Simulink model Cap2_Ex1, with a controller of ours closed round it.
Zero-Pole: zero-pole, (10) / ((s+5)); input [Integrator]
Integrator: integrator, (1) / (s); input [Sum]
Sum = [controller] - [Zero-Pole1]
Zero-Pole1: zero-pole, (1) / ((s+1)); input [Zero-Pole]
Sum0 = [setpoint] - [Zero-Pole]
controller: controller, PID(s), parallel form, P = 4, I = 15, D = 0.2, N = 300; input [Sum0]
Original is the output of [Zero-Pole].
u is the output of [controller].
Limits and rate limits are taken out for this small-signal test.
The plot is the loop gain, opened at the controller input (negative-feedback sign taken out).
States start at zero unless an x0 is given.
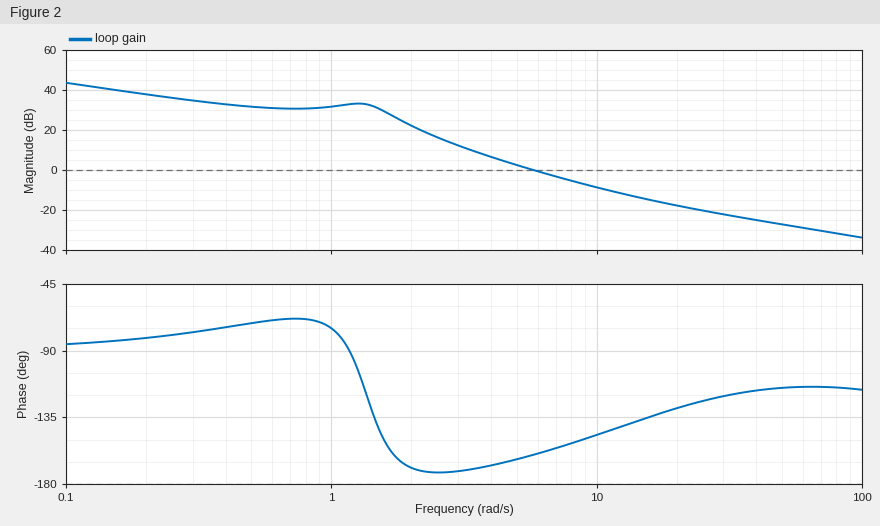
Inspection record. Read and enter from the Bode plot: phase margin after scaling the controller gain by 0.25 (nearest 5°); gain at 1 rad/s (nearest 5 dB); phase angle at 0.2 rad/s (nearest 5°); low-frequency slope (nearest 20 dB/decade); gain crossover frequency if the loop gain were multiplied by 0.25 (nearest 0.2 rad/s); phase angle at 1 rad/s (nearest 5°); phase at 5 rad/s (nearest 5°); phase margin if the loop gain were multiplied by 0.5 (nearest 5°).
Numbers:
10°
30 dB
-80°
-20 dB/decade
3.0 rad/s
-75°
-165°
15°
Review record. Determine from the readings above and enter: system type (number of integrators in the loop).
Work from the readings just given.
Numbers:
1
